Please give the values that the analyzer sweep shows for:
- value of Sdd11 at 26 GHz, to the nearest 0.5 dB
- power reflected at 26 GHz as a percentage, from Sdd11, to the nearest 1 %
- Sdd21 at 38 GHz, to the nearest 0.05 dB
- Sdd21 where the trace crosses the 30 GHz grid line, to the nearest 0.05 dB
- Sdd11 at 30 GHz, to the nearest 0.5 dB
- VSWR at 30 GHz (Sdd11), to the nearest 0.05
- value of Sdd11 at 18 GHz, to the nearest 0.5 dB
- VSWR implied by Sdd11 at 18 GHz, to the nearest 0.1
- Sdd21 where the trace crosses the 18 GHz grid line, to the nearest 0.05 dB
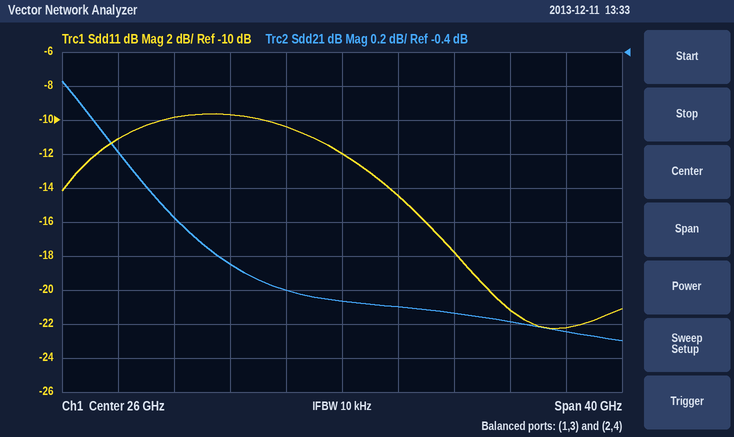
-12.0 dB
6 %
-2.00 dB
-1.90 dB
-14.5 dB
1.45
-9.5 dB
2.0
-1.65 dB
